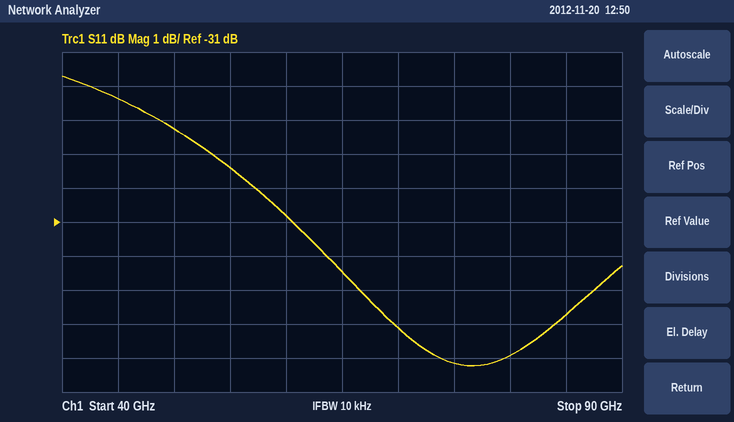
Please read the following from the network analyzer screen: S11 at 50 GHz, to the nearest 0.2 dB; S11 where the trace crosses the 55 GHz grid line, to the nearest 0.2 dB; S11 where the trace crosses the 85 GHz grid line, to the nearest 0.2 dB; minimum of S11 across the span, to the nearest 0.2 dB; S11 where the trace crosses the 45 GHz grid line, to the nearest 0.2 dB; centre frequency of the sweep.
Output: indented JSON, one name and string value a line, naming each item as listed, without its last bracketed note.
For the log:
{
  "S11 at 50 GHz, to the nearest 0.2 dB": "-28.2 dB",
  "S11 where the trace crosses the 55 GHz grid line, to the nearest 0.2 dB": "-29.4 dB",
  "S11 where the trace crosses the 85 GHz grid line, to the nearest 0.2 dB": "-33.8 dB",
  "minimum of S11 across the span, to the nearest 0.2 dB": "-35.2 dB",
  "S11 where the trace crosses the 45 GHz grid line, to the nearest 0.2 dB": "-27.4 dB",
  "centre frequency of the sweep": "65 GHz"
}
